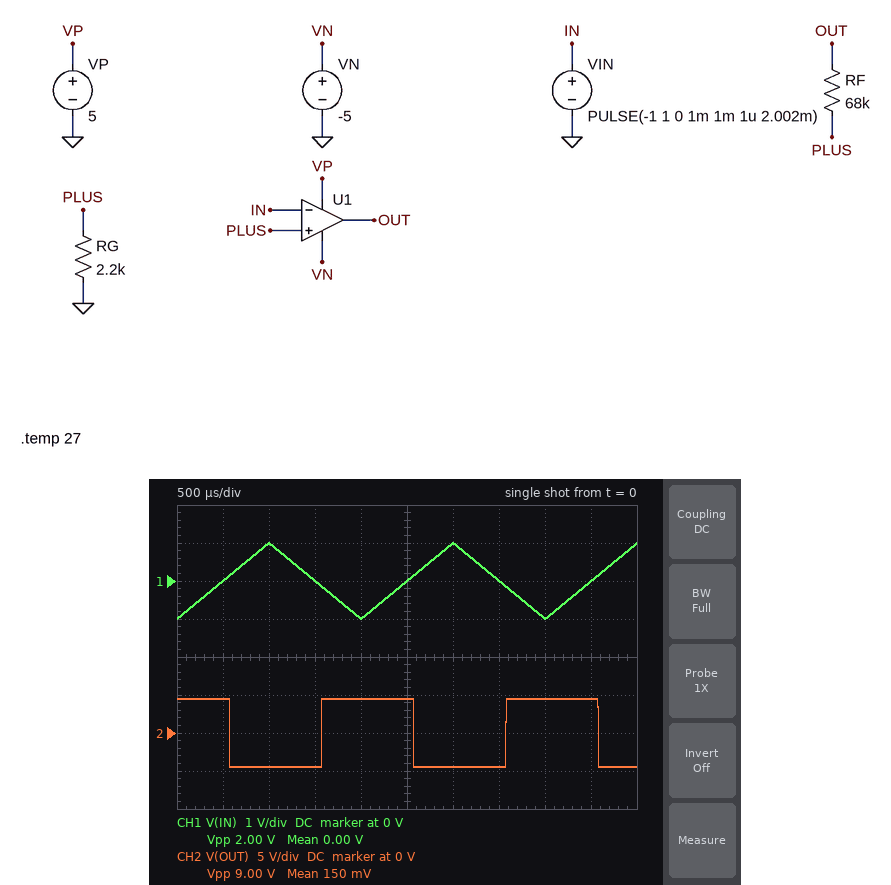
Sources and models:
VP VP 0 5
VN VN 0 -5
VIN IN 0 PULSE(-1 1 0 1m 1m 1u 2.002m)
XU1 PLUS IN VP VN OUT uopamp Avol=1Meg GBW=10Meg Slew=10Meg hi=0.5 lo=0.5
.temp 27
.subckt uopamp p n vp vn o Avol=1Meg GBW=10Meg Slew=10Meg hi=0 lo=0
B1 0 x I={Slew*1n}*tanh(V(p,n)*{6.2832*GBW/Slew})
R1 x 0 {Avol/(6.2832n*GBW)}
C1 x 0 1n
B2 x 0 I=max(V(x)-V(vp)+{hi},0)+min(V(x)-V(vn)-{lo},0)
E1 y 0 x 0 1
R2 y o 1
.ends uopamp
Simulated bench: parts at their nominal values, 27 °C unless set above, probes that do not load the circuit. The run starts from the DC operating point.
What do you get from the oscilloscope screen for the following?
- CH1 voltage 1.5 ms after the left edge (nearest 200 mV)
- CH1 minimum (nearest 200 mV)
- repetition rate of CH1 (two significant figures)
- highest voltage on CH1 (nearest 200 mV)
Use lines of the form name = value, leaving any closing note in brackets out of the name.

CH1 voltage 1.5 ms after the left edge = 0 V
CH1 minimum = -1.0 V
repetition rate of CH1 = 500 Hz
highest voltage on CH1 = 1.0 V
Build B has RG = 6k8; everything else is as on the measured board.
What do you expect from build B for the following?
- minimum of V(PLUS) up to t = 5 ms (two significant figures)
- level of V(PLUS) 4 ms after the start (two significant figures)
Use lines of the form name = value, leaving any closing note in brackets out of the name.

minimum of V(PLUS) up to t = 5 ms = -410 mV
level of V(PLUS) 4 ms after the start = 410 mV
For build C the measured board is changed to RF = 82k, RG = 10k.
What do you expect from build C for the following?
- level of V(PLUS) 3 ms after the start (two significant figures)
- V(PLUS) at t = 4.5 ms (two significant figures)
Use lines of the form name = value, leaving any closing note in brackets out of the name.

level of V(PLUS) 3 ms after the start = -490 mV
V(PLUS) at t = 4.5 ms = 490 mV
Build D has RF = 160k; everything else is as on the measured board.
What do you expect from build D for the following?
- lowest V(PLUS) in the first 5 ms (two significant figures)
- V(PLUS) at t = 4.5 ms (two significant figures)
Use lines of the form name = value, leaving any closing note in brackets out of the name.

lowest V(PLUS) in the first 5 ms = -61 mV
V(PLUS) at t = 4.5 ms = 61 mV
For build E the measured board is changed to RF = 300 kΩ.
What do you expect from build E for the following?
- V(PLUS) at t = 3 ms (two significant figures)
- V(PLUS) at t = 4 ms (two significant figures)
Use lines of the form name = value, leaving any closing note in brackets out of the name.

V(PLUS) at t = 3 ms = -33 mV
V(PLUS) at t = 4 ms = 33 mV
